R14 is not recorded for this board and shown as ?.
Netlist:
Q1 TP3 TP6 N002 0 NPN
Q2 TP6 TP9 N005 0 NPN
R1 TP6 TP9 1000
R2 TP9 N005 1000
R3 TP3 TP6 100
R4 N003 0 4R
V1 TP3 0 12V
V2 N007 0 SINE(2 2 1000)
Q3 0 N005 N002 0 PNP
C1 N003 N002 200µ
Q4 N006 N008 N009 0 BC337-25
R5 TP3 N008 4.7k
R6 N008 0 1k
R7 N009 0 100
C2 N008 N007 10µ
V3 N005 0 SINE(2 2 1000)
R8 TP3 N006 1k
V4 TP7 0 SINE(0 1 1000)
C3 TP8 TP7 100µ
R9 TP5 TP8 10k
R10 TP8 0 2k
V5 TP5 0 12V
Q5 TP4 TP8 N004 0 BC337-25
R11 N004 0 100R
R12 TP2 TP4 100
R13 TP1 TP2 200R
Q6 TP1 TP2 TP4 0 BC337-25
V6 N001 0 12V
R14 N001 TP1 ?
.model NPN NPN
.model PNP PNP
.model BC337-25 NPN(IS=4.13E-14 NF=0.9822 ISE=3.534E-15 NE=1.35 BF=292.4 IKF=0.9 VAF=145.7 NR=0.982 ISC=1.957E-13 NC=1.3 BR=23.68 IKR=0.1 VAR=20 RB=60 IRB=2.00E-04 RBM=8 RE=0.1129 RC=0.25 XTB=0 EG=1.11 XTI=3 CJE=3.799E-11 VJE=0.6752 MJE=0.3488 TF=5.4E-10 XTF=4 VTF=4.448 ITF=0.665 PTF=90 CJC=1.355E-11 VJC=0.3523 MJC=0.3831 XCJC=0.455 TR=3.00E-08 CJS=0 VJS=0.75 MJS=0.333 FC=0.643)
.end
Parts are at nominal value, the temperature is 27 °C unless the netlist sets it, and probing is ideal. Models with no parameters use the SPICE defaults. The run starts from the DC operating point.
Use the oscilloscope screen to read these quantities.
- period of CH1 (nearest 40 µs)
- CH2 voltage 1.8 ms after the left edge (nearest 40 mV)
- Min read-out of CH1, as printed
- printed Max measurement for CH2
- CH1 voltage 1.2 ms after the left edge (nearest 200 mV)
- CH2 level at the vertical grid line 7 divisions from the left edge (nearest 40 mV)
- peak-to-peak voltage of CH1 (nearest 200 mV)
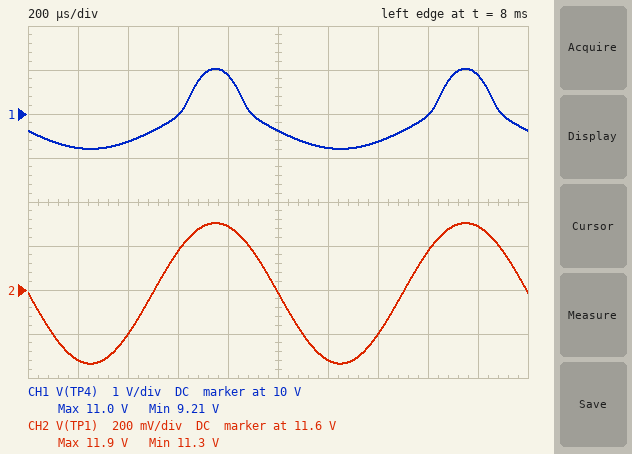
1.00 ms
11.88 V
9.21 V
11.9 V
9.2 V
11.40 V
1.8 V
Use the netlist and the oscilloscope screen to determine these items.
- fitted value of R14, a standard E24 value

33 Ω
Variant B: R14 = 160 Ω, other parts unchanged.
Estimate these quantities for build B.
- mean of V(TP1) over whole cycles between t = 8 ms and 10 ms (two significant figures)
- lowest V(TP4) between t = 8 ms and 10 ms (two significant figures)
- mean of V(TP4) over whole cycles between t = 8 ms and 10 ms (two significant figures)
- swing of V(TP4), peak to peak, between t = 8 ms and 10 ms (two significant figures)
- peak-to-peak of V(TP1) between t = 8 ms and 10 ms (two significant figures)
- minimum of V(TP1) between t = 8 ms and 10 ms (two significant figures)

10 V
6.4 V
8.2 V
4.3 V
3.1 V
8.4 V
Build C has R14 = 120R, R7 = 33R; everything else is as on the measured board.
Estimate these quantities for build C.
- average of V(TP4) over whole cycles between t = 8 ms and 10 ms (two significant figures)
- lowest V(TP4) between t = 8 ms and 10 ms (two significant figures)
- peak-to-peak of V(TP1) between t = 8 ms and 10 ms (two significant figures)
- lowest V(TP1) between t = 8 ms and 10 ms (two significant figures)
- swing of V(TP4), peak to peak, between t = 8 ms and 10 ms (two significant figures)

8.7 V
7.3 V
2.3 V
9.3 V
3.5 V
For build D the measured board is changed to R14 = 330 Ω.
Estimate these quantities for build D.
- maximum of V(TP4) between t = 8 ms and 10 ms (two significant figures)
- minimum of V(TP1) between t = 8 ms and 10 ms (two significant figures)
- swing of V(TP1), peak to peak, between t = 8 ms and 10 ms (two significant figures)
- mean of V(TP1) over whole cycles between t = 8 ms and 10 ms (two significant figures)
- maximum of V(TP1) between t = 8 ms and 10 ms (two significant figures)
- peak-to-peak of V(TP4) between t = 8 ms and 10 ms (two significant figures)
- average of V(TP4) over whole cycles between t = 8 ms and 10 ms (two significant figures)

10 V
4.7 V
6.4 V
7.9 V
11 V
7.6 V
6.1 V
